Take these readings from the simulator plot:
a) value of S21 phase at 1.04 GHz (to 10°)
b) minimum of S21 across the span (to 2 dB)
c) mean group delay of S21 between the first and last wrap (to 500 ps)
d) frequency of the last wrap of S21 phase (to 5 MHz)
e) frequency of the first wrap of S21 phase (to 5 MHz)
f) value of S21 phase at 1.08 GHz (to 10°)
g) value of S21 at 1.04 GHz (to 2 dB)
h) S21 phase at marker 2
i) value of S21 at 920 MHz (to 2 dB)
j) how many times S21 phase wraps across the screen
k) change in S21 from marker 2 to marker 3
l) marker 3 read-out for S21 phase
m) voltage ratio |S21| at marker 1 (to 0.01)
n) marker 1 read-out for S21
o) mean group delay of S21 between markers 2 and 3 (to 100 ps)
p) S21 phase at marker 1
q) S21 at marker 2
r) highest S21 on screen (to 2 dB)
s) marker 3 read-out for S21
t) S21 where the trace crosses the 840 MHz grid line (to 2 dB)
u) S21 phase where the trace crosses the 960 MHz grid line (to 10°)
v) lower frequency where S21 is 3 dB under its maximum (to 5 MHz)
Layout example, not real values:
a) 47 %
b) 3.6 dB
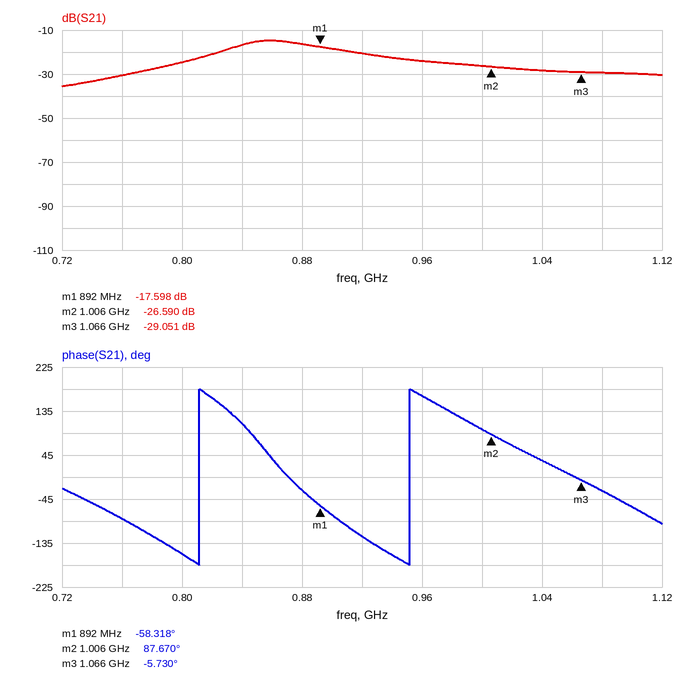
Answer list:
a) 30°
b) -36 dB
c) 7.0 ns
d) 950 MHz
e) 810 MHz
f) -30°
g) -28 dB
h) 87.670°
i) -20 dB
j) 2
k) -2.461 dB
l) -5.730°
m) 0.13
n) -17.598 dB
o) 4.3 ns
p) -58.318°
q) -26.590 dB
r) -14 dB
s) -29.051 dB
t) -16 dB
u) 170°
v) 835 MHz
